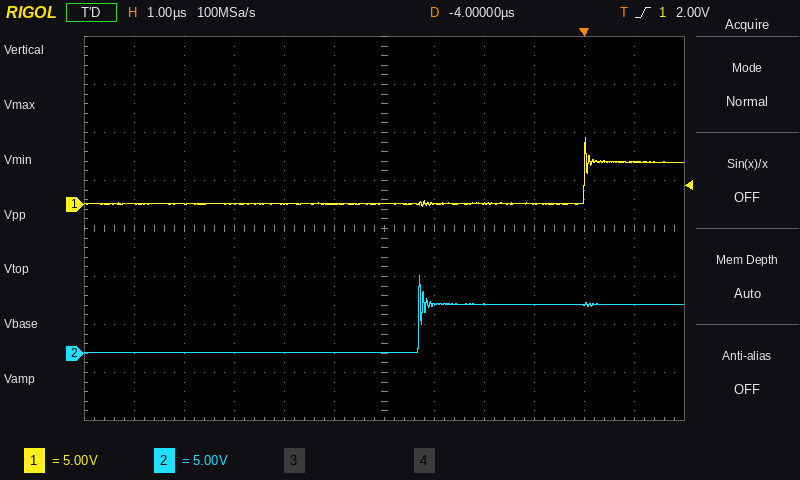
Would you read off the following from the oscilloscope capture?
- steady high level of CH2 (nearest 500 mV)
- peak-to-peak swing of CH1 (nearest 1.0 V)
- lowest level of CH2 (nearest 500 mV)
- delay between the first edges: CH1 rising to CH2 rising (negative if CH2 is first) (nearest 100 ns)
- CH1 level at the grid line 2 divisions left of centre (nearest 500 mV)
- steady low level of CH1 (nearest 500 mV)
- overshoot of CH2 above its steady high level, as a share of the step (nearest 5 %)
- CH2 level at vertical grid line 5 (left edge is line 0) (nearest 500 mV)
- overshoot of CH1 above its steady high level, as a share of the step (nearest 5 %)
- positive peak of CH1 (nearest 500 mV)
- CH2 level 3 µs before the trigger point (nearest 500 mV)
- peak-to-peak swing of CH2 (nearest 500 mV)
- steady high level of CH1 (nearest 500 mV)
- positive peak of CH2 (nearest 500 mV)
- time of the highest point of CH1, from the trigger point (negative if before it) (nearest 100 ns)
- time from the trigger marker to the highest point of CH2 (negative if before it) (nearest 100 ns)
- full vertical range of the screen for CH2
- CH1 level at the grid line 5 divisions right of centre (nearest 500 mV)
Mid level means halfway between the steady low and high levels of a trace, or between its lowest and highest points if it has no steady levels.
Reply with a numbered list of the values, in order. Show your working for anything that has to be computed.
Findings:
1. 5.0 V
2. 7.0 V
3. 0.0 V
4. -3.3 µs
5. 0.0 V
6. 0.0 V
7. 60 %
8. 0.0 V
9. 60 %
10. 7.0 V
11. 5.0 V
12. 8.0 V − (0.0 V) = 8.0 V
13. 4.5 V
14. 8.0 V
15. 0.0 µs
16. -3.3 µs
17. 40 V
18. 4.5 V
